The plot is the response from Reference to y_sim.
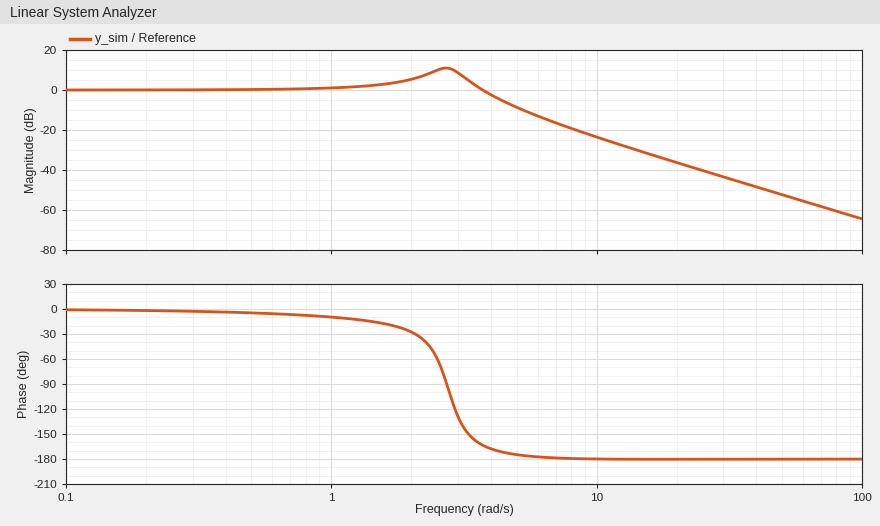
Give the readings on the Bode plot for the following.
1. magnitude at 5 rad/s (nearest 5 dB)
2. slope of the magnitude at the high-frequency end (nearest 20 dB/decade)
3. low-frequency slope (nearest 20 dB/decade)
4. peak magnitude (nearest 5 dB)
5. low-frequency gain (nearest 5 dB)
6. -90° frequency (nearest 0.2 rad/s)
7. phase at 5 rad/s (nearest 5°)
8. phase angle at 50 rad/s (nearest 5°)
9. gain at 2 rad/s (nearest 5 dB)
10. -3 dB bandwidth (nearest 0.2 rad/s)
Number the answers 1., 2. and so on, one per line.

1. -10 dB
2. -40 dB/decade
3. 0 dB/decade
4. 10 dB
5. 0 dB
6. 2.8 rad/s
7. -175°
8. -180°
9. 5 dB
10. 4.0 rad/s
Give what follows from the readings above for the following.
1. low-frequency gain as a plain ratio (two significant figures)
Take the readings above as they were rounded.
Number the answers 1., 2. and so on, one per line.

1. 1.0
